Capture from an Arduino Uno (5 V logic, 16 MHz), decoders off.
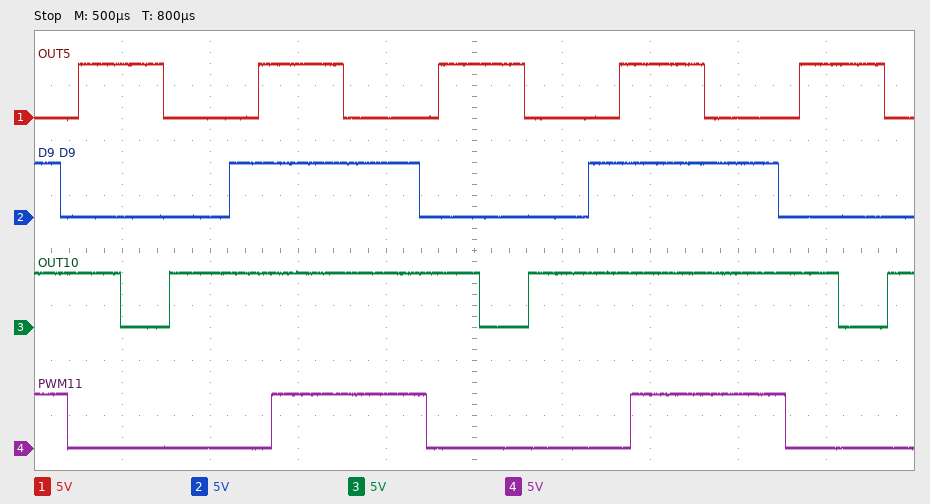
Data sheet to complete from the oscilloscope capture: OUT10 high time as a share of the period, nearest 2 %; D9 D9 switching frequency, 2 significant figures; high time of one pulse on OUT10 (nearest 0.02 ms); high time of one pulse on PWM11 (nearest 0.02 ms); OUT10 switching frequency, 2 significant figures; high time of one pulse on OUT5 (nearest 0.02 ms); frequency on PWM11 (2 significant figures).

86 %
490 Hz
1.76 ms
0.88 ms
490 Hz
0.48 ms
490 Hz
